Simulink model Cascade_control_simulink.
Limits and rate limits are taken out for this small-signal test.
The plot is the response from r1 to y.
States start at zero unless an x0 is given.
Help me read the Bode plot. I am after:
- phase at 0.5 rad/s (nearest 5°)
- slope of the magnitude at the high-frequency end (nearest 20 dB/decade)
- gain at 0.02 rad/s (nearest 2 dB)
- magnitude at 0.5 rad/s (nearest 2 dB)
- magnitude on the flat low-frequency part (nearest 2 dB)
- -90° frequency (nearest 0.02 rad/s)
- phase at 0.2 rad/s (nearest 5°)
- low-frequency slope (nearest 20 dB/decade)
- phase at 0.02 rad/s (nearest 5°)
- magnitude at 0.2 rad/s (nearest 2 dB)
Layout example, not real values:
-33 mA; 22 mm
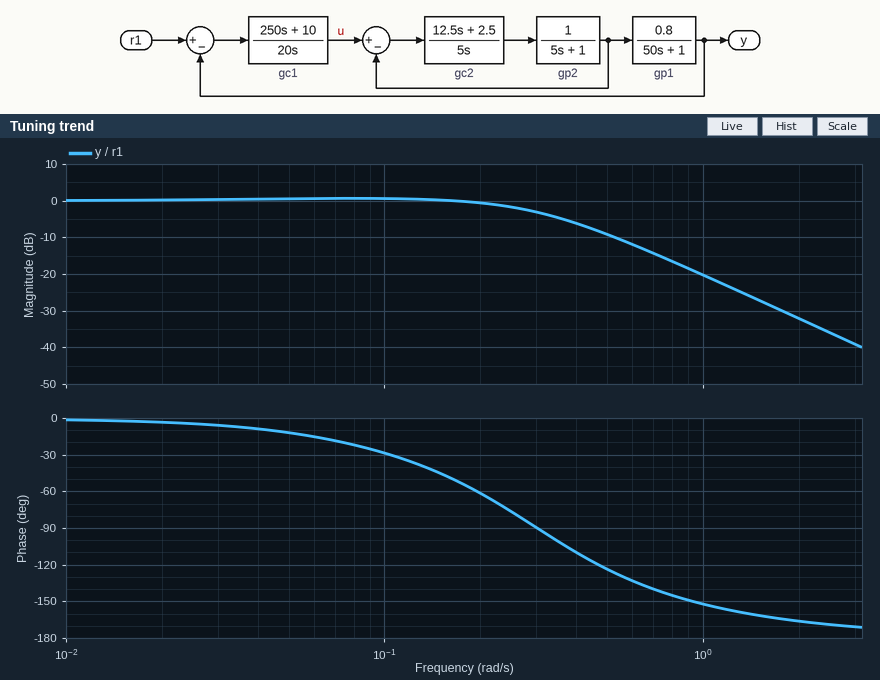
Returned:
-125°; -40 dB/decade; 0 dB; -10 dB; 0 dB; 0.30 rad/s; -60°; 0 dB/decade; -5°; 0 dB
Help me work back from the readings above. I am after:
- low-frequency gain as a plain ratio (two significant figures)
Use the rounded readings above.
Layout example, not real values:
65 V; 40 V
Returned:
1.0
